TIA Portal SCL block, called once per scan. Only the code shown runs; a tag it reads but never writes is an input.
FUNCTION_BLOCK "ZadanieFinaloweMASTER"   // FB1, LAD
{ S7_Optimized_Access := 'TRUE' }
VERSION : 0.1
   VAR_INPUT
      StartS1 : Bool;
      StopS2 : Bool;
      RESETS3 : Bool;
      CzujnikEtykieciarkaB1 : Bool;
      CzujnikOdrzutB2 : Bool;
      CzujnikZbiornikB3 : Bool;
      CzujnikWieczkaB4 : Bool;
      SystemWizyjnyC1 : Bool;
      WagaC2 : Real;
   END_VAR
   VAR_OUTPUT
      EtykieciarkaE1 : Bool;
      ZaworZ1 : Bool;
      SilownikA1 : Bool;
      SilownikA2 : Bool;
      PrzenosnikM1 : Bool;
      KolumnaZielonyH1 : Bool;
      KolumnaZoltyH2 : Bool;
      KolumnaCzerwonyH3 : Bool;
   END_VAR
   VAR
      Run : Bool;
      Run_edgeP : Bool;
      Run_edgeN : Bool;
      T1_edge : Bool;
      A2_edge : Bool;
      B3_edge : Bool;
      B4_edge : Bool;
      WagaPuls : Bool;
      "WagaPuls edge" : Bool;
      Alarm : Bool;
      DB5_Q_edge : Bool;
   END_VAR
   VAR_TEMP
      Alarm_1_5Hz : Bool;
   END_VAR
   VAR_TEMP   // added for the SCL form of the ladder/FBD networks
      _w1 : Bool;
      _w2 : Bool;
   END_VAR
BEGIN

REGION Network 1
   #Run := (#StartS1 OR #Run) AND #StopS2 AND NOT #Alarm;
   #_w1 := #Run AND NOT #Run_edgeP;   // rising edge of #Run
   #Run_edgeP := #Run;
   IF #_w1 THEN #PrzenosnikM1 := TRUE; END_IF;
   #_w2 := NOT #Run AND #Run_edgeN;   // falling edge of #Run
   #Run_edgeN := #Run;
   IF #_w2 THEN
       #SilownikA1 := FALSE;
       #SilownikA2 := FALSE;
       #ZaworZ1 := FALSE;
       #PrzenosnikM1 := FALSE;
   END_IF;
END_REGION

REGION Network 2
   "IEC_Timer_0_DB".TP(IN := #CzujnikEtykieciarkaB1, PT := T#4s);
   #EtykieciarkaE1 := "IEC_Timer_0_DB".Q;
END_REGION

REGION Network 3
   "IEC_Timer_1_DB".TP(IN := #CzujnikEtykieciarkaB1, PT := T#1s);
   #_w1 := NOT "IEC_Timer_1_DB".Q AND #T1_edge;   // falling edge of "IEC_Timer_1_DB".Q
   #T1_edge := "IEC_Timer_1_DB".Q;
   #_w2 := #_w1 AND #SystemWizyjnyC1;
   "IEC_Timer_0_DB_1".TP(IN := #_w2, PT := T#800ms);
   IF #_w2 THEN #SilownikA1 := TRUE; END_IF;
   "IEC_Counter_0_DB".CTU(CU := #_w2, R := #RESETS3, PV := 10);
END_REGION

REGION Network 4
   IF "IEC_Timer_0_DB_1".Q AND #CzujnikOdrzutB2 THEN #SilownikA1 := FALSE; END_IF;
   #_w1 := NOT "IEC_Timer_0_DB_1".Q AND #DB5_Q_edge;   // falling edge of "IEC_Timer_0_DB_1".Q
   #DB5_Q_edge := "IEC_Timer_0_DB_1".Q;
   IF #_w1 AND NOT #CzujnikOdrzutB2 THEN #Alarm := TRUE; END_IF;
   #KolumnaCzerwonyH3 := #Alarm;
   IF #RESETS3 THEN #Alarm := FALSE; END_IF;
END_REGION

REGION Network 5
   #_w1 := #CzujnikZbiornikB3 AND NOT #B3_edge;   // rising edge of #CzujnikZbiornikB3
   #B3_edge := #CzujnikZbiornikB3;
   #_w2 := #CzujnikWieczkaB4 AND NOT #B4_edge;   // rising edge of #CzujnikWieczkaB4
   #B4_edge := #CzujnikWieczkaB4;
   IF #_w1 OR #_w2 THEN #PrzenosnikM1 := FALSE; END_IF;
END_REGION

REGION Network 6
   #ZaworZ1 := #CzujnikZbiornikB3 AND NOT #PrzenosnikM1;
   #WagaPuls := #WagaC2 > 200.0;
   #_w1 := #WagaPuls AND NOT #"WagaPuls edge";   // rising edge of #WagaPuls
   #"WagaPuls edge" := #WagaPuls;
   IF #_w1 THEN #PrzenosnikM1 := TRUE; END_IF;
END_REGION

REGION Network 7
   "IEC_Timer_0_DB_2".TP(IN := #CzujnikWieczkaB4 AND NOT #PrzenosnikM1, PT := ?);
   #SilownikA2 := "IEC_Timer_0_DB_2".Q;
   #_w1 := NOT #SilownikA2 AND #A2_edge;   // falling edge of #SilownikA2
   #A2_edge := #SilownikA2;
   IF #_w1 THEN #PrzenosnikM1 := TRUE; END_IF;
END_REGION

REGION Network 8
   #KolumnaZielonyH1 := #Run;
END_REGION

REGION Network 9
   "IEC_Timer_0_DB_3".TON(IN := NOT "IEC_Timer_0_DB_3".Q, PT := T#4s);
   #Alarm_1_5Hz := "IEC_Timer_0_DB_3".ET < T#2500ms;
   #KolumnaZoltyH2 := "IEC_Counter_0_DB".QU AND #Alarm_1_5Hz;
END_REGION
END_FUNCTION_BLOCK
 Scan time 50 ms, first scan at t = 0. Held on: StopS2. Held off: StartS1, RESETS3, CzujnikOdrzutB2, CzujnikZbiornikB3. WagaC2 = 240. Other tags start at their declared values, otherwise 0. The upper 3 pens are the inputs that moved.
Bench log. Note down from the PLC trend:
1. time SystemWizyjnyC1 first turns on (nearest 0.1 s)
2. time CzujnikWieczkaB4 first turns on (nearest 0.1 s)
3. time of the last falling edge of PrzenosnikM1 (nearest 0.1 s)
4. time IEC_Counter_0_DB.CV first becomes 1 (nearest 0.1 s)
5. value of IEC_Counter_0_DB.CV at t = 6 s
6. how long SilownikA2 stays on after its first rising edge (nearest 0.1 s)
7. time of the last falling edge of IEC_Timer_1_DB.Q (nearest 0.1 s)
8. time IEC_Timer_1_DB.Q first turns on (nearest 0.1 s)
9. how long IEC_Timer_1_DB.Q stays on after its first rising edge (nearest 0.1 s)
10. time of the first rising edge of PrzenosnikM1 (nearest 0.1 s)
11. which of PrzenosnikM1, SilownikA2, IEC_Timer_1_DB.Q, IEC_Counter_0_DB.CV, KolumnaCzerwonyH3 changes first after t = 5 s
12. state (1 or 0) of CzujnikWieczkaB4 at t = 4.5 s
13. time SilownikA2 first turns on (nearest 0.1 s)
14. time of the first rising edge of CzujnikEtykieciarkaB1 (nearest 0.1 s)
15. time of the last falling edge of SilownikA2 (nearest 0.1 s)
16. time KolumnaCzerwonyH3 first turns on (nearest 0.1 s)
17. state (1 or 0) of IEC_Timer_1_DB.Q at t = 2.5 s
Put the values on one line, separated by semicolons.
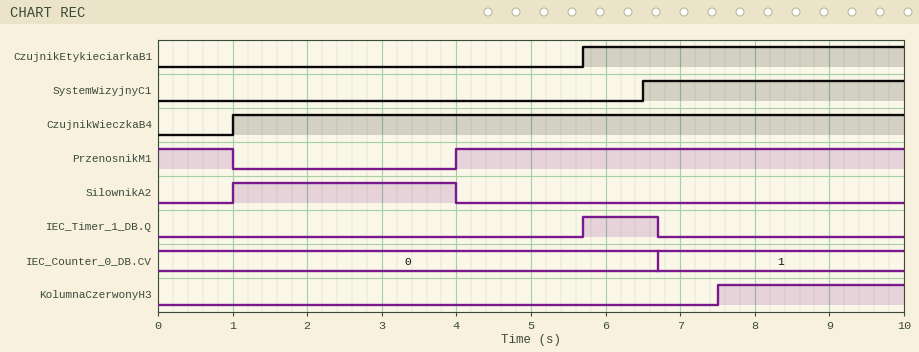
6.5 s; 1.0 s; 1.0 s; 6.7 s; 0; 3.0 s; 6.7 s; 5.7 s; 1.0 s; 4.0 s; IEC_Timer_1_DB.Q; 1; 1.0 s; 5.7 s; 4.0 s; 7.5 s; 0
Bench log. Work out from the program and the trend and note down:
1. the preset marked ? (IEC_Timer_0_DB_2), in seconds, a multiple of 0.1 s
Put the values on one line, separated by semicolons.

3.0 s
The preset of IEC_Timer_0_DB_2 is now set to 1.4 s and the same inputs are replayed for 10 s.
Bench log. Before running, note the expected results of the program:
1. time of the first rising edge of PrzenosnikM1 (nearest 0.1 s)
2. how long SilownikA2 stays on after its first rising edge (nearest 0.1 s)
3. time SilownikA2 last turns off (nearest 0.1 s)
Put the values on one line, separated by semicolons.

2.4 s; 1.4 s; 2.4 s
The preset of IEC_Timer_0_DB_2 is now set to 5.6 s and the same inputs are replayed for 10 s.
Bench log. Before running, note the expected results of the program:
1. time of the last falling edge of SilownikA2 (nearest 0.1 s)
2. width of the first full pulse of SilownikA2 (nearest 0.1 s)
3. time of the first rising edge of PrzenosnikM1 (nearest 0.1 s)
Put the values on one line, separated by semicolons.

6.6 s; 5.6 s; 6.6 s
